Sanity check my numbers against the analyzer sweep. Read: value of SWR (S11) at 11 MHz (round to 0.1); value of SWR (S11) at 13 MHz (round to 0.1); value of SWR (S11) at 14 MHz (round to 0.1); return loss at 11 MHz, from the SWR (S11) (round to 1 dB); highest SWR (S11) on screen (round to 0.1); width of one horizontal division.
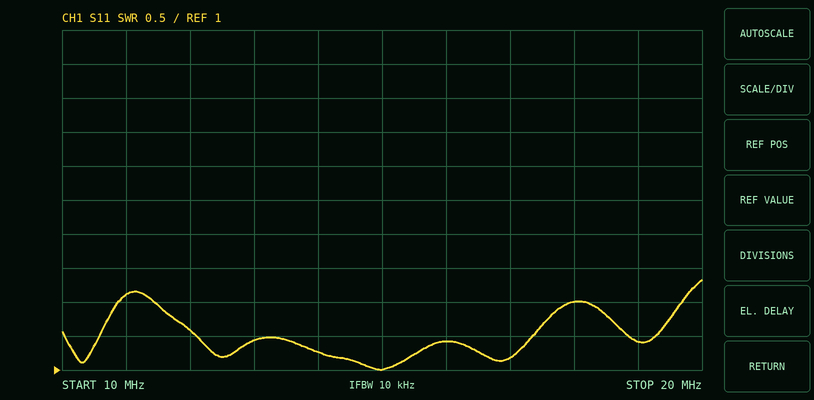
2.1
1.4
1.3
9 dB
2.3
1 MHz
